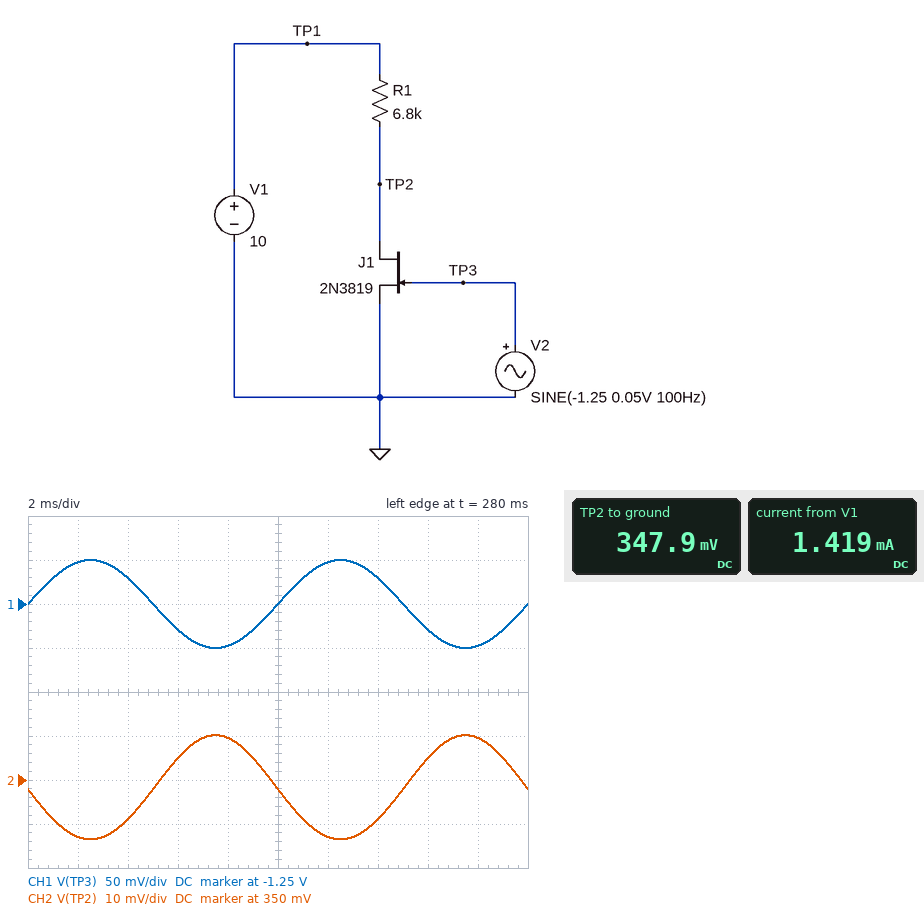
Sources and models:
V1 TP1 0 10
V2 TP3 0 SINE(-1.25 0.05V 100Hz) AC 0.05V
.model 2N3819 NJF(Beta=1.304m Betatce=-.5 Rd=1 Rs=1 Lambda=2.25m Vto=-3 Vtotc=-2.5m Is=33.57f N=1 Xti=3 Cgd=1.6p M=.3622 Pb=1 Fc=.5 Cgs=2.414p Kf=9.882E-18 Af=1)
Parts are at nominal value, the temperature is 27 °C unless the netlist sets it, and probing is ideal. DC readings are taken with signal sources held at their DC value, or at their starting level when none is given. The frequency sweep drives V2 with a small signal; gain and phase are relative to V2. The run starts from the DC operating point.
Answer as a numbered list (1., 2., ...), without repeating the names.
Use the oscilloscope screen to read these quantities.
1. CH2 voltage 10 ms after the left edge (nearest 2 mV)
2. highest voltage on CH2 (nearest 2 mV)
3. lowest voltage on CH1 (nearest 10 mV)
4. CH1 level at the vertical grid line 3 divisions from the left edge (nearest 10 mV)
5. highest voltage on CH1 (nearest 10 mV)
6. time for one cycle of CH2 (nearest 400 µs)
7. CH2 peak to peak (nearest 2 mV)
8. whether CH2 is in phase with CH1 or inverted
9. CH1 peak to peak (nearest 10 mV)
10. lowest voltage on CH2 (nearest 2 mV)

1. 348 mV
2. 360 mV
3. -1.30 V
4. -1.28 V
5. -1.20 V
6. 10.0 ms
7. 24 mV
8. inverted
9. 100 mV
10. 336 mV
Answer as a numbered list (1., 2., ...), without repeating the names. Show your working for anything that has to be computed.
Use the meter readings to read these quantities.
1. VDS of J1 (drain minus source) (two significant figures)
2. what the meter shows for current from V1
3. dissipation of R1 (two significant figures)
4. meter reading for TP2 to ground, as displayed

1. 347.9 mV = 350 mV
2. 1.419 mA
3. (10 V - 347.9 mV)^2 / 6.8 kΩ = 14 mW
4. 347.9 mV
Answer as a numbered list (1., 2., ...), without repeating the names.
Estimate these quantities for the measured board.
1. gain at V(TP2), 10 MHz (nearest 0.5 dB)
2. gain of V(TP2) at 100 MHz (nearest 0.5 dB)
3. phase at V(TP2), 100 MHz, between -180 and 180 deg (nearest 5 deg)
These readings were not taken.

1. -12.5 dB
2. -11.0 dB
3. 135 deg
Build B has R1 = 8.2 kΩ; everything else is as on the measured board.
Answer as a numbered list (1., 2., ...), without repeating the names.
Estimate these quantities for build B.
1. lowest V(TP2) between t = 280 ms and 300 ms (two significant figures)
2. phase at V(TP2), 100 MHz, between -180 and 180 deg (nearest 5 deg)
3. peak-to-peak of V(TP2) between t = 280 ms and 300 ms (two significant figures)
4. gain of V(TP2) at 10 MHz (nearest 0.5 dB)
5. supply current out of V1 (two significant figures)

1. 280 mV
2. 130 deg
3. 19 mV
4. -14.5 dB
5. 1.2 mA
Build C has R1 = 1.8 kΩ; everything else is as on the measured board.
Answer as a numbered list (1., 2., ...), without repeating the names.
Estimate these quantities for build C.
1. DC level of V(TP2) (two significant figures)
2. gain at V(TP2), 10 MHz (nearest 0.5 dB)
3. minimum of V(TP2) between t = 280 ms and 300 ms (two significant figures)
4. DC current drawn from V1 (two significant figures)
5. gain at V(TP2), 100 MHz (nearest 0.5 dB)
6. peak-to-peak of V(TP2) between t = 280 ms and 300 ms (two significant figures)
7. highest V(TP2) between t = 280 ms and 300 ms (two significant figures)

1. 2.8 V
2. 18.0 dB
3. 2.4 V
4. 4.0 mA
5. 16.0 dB
6. 810 mV
7. 3.2 V
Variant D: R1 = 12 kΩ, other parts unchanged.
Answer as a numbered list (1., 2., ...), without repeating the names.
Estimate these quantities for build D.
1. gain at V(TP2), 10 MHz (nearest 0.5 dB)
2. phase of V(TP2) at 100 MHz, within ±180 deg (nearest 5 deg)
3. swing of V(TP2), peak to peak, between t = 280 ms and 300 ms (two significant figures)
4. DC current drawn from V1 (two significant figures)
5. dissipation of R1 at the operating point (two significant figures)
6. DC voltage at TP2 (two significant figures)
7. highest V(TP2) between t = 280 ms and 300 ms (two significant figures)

1. -18.5 dB
2. 120 deg
3. 12 mV
4. 820 µA
5. 8.0 mW
6. 190 mV
7. 200 mV
